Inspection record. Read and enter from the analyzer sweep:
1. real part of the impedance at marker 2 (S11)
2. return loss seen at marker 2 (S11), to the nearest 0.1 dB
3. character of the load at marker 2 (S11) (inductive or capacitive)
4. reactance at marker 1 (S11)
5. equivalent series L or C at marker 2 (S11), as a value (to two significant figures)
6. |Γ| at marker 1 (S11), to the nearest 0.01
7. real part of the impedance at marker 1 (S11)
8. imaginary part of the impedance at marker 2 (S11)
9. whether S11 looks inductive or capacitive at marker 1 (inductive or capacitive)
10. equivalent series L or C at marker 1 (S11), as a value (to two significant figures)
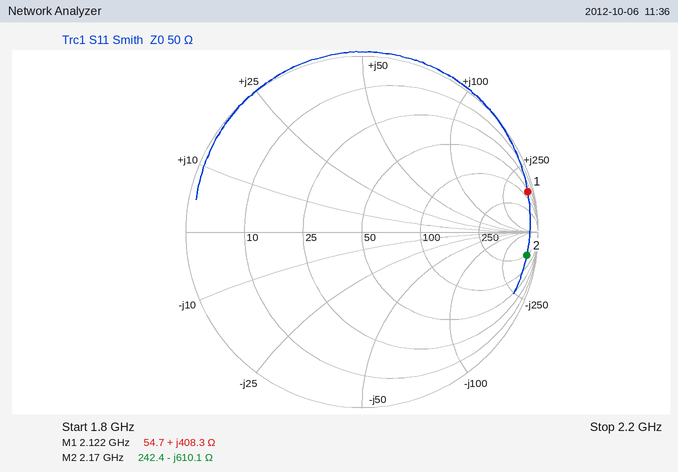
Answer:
242.4 Ω
0.5 dB
capacitive
+408.3 Ω
120 fF
0.97
54.7 Ω
-610.1 Ω
inductive
31 nH
